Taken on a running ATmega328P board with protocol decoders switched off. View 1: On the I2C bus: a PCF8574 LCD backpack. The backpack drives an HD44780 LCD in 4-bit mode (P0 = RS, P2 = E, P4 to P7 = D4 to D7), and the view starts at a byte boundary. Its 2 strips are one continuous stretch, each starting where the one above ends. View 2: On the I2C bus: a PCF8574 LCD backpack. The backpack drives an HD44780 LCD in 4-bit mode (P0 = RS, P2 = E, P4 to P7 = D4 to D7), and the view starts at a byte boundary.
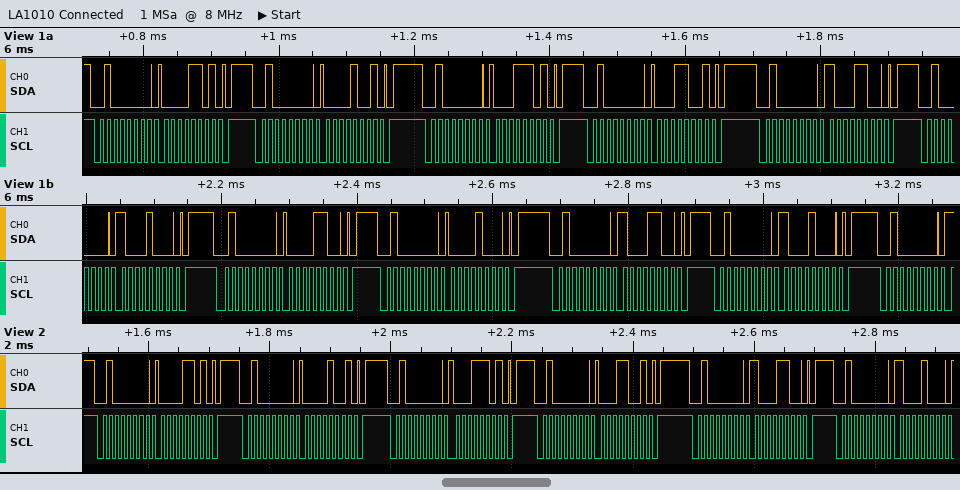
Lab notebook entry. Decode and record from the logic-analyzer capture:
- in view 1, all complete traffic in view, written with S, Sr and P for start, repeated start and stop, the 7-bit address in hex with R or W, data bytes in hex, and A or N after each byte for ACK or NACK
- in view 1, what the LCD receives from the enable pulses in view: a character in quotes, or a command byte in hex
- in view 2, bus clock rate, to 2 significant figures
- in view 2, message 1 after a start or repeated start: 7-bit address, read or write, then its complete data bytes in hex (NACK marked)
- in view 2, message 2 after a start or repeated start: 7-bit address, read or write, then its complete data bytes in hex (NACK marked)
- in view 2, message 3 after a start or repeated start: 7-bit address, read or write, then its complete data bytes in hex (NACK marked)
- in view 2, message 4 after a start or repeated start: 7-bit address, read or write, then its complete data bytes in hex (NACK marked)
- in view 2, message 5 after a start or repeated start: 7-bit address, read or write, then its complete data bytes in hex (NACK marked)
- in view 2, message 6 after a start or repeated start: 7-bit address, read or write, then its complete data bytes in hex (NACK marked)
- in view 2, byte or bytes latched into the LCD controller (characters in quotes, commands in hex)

S 20W A 0D A P S 20W A 09 A P S 20W A 1D A P S 20W A 19 A P S 20W A 8C A P S 20W A 88 A P S 20W A 0C A P S 20W A 08 A P S 20W A 8C A P S 20W A 88 A P S 20W A
data 0x01 0x80
100 kHz
0x20 write: 0D
0x20 write: 09
0x20 write: 1D
0x20 write: 19
0x20 write: 8C
0x20 write: 88
data 0x01
